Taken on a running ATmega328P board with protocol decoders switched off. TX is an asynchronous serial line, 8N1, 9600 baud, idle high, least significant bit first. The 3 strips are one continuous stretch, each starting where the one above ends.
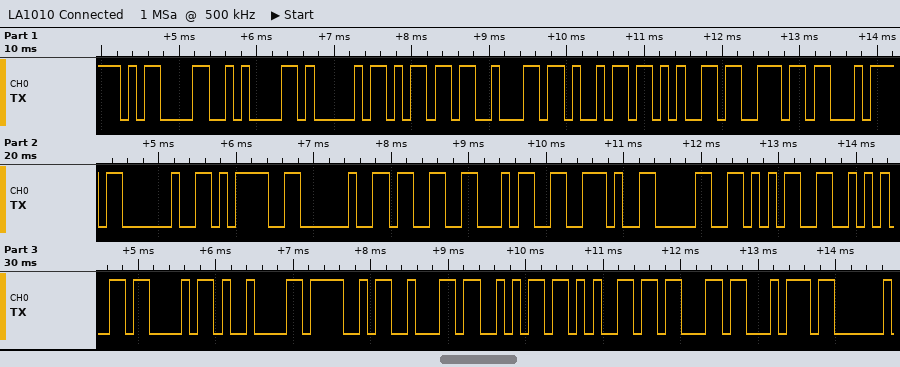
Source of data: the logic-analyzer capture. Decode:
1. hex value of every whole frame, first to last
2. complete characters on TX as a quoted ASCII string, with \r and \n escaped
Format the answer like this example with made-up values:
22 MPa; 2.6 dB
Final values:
0x0D 0x0A 0x41 0x6D 0x62 0x69 0x65 0x6E 0x74 0x20 0x3D 0x20 0x33 0x34 0x2E 0x30 0x35 0x2A 0x43 0x09 0x4F 0x62 0x6A 0x65 0x63 0x74; "\r\nAmbient = 34.05*C\tObject"
